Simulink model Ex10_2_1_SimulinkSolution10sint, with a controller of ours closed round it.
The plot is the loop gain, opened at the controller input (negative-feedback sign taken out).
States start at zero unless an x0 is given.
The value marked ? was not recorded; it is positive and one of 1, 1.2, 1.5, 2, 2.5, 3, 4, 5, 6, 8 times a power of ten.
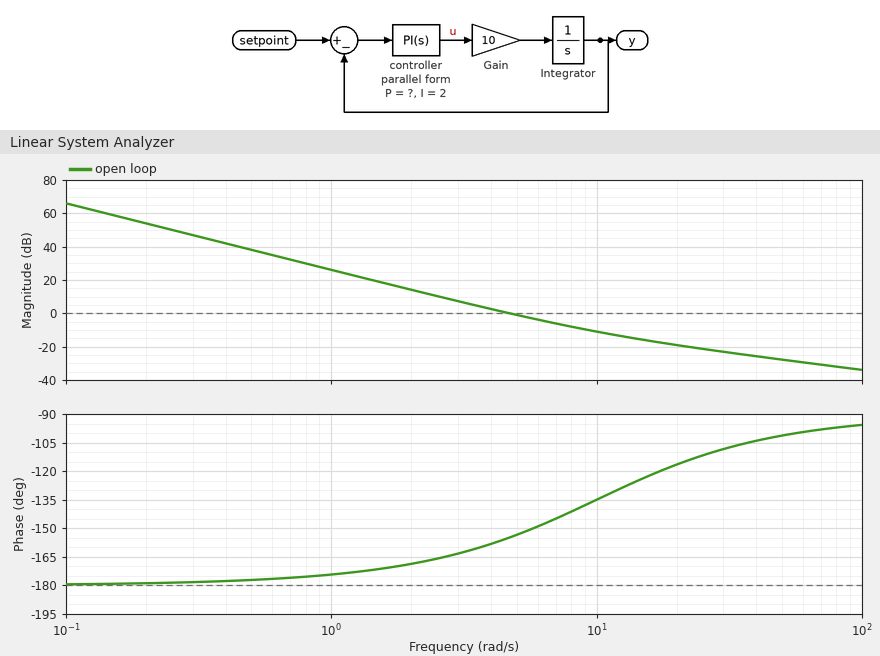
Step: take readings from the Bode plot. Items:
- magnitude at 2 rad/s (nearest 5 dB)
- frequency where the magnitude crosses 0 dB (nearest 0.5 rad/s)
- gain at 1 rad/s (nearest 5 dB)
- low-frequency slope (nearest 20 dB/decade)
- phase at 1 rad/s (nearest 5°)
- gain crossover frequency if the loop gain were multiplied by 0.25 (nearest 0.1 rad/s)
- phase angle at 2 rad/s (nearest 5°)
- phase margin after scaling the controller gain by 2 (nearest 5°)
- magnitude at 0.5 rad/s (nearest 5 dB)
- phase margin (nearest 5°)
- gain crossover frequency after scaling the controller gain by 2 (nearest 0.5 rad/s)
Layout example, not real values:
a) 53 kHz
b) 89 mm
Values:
a) 15 dB
b) 4.5 rad/s
c) 25 dB
d) -40 dB/decade
e) -175°
f) 2.3 rad/s
g) -170°
h) 35°
i) 40 dB
j) 25°
k) 7.0 rad/s
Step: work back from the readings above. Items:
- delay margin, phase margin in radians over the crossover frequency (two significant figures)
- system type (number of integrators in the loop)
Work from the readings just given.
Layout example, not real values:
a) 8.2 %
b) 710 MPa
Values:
a) 0.097 s
b) 2
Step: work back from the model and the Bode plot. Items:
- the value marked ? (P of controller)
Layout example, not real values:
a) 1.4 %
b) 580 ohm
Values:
a) 0.2
